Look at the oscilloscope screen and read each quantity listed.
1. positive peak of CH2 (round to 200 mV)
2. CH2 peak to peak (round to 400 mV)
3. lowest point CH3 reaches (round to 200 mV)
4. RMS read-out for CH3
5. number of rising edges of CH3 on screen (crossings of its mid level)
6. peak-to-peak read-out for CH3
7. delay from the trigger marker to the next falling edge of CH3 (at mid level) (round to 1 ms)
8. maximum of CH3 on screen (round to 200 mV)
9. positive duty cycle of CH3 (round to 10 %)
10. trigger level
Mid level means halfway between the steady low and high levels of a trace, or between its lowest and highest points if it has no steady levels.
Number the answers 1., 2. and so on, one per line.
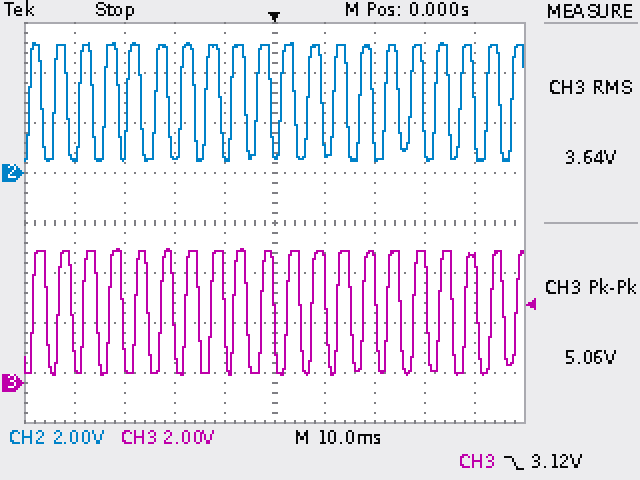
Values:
1. 5.2 V
2. 4.8 V
3. 400 mV
4. 3.64 V
5. 20
6. 5.06 V
7. 5 ms
8. 5.4 V
9. 50 %
10. 3.12 V
